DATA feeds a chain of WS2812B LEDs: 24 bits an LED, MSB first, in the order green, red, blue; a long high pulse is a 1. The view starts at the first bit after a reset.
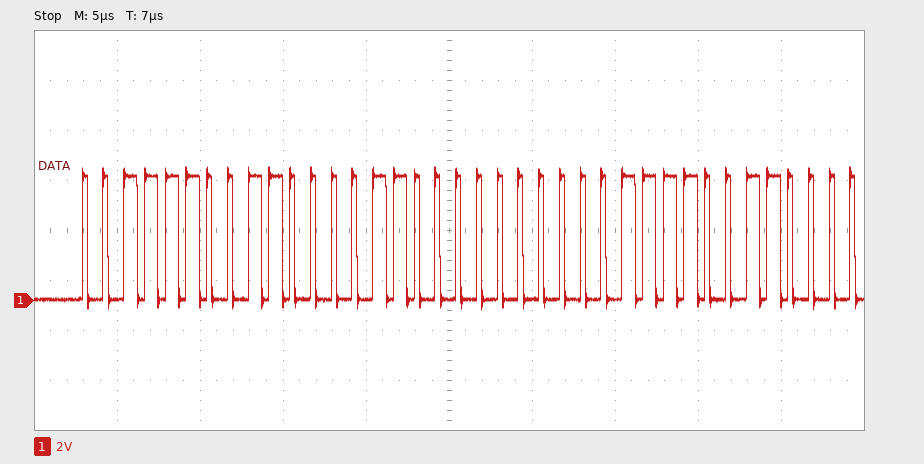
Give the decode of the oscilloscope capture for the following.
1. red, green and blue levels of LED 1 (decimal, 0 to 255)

195, 60, 0
